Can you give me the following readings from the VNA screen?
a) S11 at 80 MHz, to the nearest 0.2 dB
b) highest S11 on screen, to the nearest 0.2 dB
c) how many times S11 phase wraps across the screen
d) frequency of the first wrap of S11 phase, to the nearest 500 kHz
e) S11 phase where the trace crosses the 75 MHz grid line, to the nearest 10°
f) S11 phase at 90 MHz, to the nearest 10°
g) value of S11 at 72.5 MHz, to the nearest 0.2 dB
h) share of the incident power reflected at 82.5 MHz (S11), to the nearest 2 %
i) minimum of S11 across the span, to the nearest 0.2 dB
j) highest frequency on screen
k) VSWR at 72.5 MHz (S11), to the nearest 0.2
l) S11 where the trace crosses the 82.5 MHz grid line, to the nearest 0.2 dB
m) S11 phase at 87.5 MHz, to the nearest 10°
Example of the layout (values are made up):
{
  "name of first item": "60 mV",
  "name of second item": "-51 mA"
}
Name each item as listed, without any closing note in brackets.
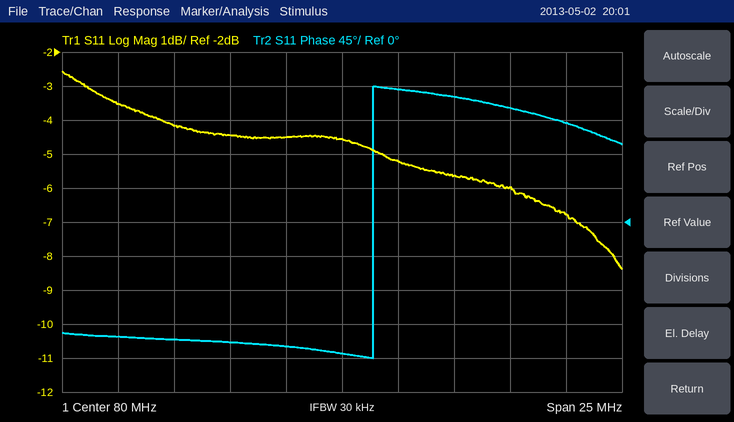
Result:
{
  "S11 at 80 MHz, to the nearest 0.2 dB": "-4.6 dB",
  "highest S11 on screen, to the nearest 0.2 dB": "-2.6 dB",
  "how many times S11 phase wraps across the screen": "1",
  "frequency of the first wrap of S11 phase, to the nearest 500 kHz": "81.5 MHz",
  "S11 phase where the trace crosses the 75 MHz grid line, to the nearest 10°": "-160°",
  "S11 phase at 90 MHz, to the nearest 10°": "130°",
  "value of S11 at 72.5 MHz, to the nearest 0.2 dB": "-4.2 dB",
  "share of the incident power reflected at 82.5 MHz (S11), to the nearest 2 %": "30 %",
  "minimum of S11 across the span, to the nearest 0.2 dB": "-8.4 dB",
  "highest frequency on screen": "92.5 MHz",
  "VSWR at 72.5 MHz (S11), to the nearest 0.2": "4.2",
  "S11 where the trace crosses the 82.5 MHz grid line, to the nearest 0.2 dB": "-5.2 dB",
  "S11 phase at 87.5 MHz, to the nearest 10°": "150°"
}
